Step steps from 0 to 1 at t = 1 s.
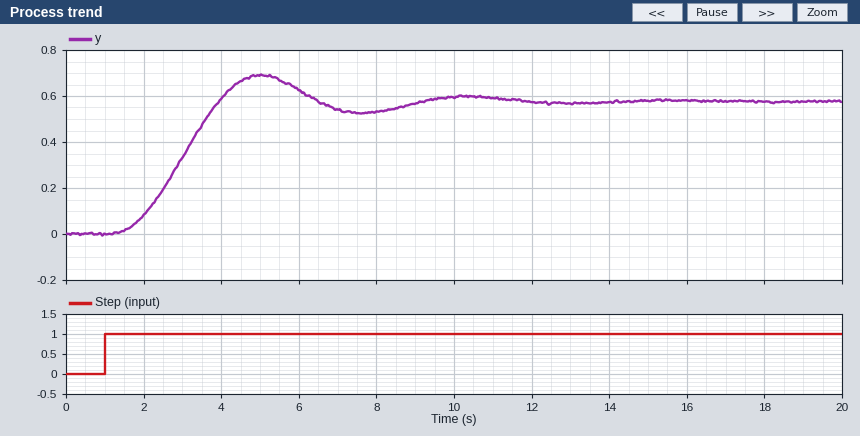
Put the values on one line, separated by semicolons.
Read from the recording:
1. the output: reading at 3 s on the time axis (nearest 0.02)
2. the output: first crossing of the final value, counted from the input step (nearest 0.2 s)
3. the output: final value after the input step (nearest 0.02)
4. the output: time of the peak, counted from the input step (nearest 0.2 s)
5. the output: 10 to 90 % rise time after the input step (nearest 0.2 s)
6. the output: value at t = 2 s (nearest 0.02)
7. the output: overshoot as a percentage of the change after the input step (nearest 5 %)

0.34; 3.0 s; 0.58; 4.0 s; 1.8 s; 0.08; 20 %
